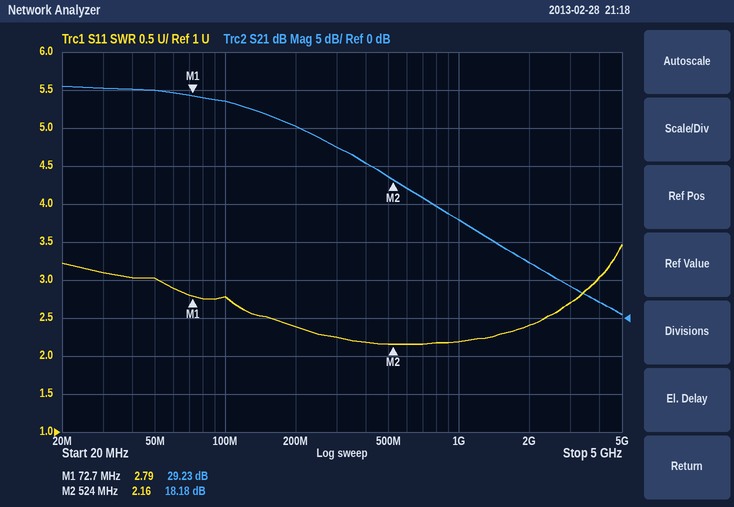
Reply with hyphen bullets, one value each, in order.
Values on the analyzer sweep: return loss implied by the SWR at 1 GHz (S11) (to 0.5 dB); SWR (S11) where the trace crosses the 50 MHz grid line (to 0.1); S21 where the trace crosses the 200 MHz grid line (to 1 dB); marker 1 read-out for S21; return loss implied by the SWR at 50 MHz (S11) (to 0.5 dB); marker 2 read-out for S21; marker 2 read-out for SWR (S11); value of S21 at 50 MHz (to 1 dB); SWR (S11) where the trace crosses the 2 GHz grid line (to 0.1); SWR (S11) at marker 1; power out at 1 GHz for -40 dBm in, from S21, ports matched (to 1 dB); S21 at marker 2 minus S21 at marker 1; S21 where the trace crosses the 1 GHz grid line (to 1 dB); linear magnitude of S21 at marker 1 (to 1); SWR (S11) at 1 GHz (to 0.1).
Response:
- 8.5 dB
- 3.0
- 25 dB
- 29.23 dB
- 6.0 dB
- 18.18 dB
- 2.16
- 30 dB
- 2.4
- 2.79
- -27 dBm
- -11.05 dB
- 13 dB
- 29
- 2.2
